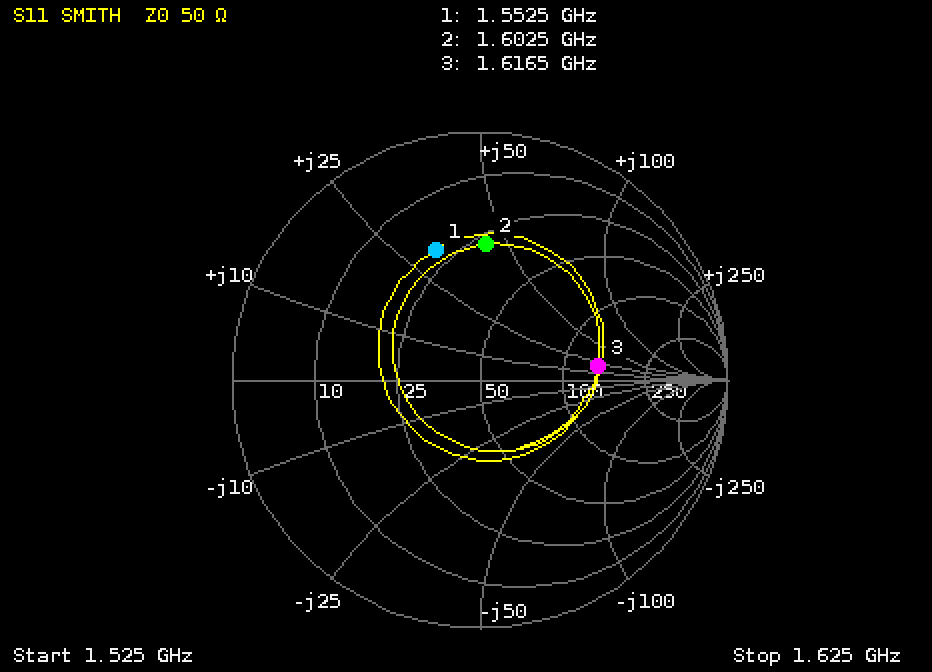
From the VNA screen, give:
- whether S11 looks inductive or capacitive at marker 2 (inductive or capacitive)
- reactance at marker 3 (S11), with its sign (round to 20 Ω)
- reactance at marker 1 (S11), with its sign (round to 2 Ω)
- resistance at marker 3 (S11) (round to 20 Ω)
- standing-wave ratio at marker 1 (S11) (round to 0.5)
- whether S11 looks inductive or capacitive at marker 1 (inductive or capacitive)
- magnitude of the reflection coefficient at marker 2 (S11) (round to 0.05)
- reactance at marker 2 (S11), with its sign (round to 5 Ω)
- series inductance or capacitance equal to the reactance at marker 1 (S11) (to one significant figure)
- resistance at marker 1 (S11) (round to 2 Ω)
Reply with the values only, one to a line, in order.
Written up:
inductive
+20 Ω
+32 Ω
140 Ω
3.5
inductive
0.55
+45 Ω
3 nH
20 Ω
